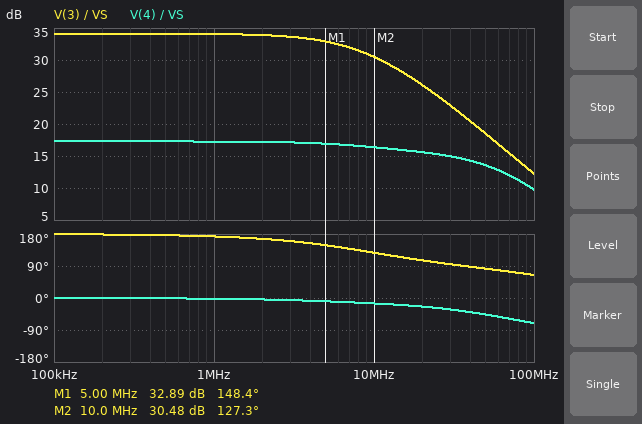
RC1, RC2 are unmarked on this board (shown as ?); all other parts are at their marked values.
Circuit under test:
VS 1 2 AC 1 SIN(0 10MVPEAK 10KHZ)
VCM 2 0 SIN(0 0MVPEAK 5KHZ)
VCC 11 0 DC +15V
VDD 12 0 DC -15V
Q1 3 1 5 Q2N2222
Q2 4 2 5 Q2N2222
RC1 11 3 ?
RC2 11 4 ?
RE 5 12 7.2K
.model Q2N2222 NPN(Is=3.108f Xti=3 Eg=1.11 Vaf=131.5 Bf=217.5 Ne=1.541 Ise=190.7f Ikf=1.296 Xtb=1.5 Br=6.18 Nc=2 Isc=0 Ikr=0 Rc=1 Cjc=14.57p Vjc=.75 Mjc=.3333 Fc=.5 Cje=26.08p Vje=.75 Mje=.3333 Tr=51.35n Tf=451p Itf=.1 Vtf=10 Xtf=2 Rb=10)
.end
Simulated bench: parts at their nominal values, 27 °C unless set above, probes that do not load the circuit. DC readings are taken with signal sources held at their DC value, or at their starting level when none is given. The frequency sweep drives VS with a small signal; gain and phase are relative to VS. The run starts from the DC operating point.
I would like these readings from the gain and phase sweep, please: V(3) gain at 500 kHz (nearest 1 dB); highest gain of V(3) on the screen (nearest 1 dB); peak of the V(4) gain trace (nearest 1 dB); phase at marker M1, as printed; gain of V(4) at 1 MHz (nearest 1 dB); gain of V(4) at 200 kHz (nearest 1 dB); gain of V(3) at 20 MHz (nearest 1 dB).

34 dB
34 dB
17 dB
148.4 deg
17 dB
17 dB
26 dB
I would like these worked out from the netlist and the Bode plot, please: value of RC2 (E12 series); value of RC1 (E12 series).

390 Ω
2.7 kΩ
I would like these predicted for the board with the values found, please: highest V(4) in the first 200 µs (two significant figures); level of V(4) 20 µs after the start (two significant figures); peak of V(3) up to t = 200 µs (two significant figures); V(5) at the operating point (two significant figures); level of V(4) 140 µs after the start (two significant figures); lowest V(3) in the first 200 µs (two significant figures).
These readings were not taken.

15 V
15 V
13 V
-680 mV
15 V
12 V
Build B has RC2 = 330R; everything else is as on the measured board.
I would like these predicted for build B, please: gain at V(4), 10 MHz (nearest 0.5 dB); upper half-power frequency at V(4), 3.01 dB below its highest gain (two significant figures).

15.0 dB
46 MHz
